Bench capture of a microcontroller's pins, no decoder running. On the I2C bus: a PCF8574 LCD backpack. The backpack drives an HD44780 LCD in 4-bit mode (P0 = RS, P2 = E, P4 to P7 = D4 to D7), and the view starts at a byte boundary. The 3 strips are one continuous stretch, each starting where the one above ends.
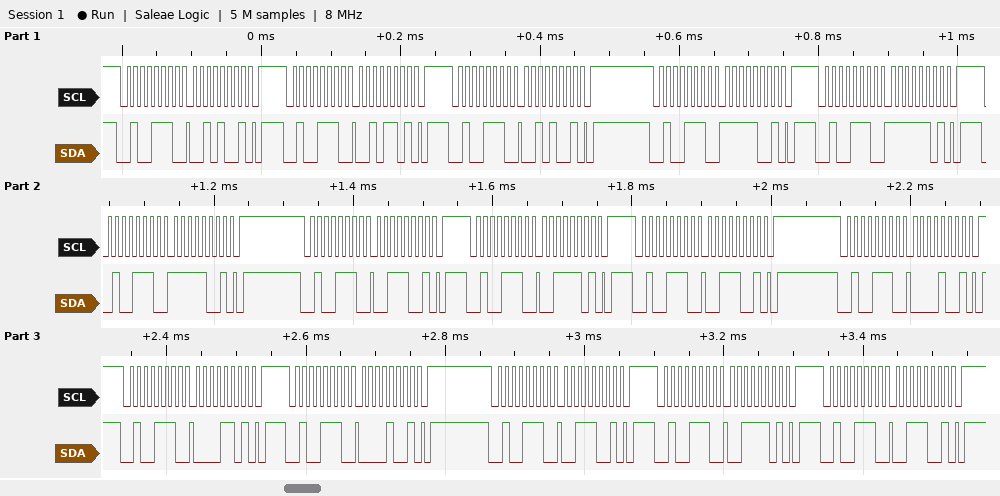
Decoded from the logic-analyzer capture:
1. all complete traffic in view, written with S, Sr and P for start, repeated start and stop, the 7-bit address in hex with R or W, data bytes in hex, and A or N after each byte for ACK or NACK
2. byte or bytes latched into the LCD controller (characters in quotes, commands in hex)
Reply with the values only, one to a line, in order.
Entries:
S 27W A 29 A P S 27W A 2D A P S 27W A 29 A P S 27W A F9 A P S 27W A FD A P S 27W A F9 A P S 27W A 39 A P S 27W A 3D A P S 27W A 39 A P S 27W A 09 A P S 27W A 0D A P S 27W A 09 A P S 27W A 39 A P S 27W A 3D A P S 27W A 39 A P
'/' '0'
